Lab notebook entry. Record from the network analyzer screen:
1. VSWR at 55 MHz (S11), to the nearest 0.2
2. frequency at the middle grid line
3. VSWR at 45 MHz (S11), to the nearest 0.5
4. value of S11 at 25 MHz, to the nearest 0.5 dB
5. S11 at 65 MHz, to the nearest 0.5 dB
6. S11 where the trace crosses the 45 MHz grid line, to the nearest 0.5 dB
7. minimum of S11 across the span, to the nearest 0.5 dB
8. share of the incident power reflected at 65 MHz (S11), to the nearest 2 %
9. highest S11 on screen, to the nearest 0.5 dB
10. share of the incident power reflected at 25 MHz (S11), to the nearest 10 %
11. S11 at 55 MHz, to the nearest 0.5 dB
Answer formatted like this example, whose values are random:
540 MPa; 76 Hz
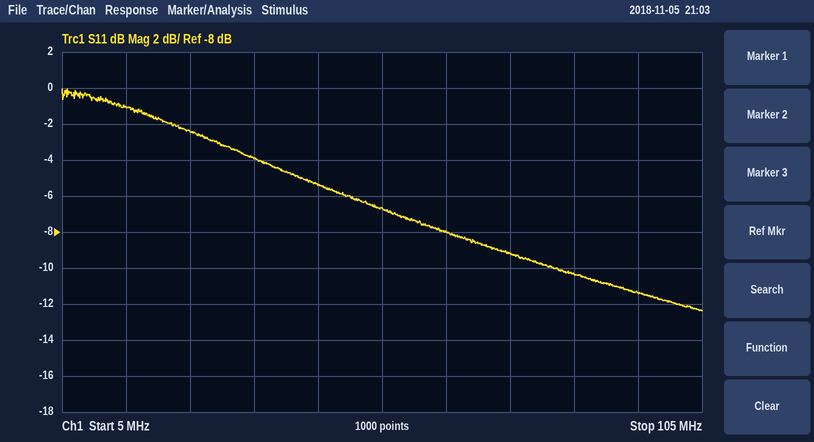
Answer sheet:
2.8; 55 MHz; 3.5; -2.5 dB; -8.0 dB; -5.5 dB; -12.5 dB; 16 %; 0.0 dB; 60 %; -6.5 dB
